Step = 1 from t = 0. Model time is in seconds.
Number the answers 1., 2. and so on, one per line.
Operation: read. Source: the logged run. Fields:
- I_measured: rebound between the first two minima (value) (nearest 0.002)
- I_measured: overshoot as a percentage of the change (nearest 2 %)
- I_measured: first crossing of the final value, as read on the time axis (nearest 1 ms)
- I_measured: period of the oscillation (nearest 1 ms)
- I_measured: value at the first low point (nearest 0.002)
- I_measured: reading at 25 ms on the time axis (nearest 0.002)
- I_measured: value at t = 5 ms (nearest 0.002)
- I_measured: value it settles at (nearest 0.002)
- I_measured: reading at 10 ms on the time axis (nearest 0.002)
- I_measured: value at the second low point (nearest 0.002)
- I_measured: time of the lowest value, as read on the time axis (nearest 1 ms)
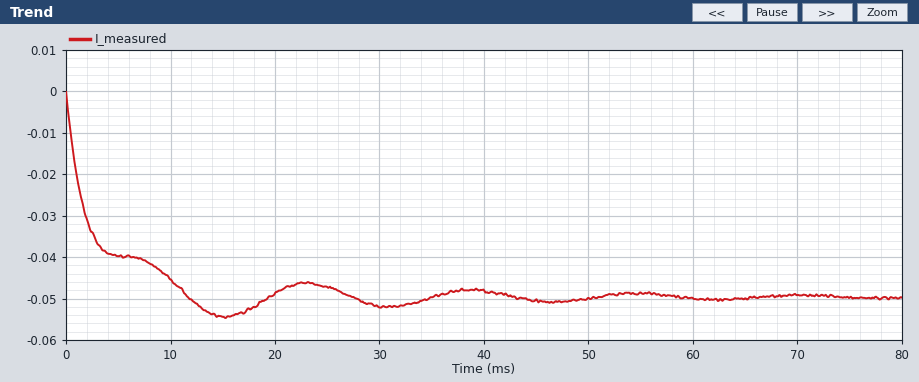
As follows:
1. -0.046
2. 10 %
3. 12 ms
4. 16 ms
5. -0.054
6. -0.048
7. -0.040
8. -0.050
9. -0.046
10. -0.052
11. 15 ms
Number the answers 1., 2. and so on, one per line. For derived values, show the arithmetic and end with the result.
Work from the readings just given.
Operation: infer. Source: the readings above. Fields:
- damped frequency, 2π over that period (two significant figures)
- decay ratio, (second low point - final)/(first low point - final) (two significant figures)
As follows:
1. 2π / 16 = 0.39 rad/ms
2. (-0.052 - (-0.05)) / (-0.054 - (-0.05)) = 0.50
